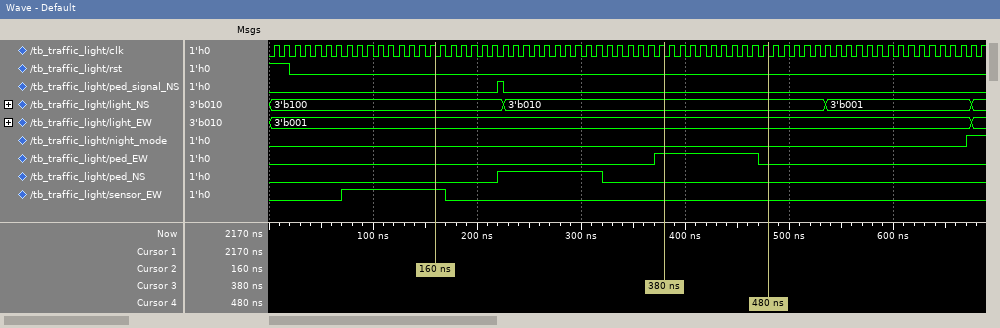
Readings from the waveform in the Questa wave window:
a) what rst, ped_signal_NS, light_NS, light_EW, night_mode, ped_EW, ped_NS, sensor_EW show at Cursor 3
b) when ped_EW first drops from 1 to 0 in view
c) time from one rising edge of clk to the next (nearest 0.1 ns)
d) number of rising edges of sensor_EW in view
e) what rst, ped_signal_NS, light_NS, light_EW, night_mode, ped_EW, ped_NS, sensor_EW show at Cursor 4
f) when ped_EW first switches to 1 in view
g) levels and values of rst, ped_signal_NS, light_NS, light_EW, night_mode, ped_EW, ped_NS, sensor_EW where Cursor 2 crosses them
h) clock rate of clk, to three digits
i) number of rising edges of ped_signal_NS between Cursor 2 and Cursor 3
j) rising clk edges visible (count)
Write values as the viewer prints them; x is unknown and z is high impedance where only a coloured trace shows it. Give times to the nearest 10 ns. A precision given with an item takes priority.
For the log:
rst=0, ped_signal_NS=0, light_NS=3'b010, light_EW=3'b001, night_mode=0, ped_EW=1, ped_NS=0, sensor_EW=0
470 ns
10 ns
1
rst=0, ped_signal_NS=0, light_NS=3'b010, light_EW=3'b001, night_mode=0, ped_EW=0, ped_NS=0, sensor_EW=0
370 ns
rst=0, ped_signal_NS=0, light_NS=3'b100, light_EW=3'b001, night_mode=0, ped_EW=0, ped_NS=0, sensor_EW=1
100 MHz
1
69
